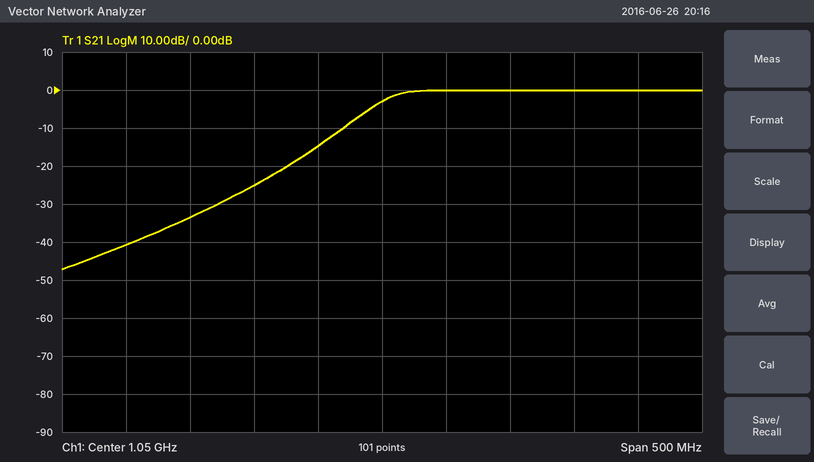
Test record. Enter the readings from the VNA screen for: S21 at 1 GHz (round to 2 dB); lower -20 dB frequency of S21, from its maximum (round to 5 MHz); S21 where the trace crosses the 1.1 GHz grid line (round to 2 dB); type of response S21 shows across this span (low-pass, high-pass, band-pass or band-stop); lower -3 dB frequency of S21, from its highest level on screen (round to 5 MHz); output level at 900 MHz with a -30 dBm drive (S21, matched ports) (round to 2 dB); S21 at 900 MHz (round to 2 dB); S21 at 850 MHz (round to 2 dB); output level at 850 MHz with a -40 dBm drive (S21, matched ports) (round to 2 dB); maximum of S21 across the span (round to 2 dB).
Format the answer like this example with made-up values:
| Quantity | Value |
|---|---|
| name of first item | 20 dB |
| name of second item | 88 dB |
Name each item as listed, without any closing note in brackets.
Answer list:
| Quantity | Value |
|---|---|
| S21 at 1 GHz | -14 dB |
| lower -20 dB frequency of S21, from its maximum | 975 MHz |
| S21 where the trace crosses the 1.1 GHz grid line | 0 dB |
| type of response S21 shows across this span | high-pass |
| lower -3 dB frequency of S21, from its highest level on screen | 1.050 GHz |
| output level at 900 MHz with a -30 dBm drive (S21, matched ports) | -64 dBm |
| S21 at 900 MHz | -34 dB |
| S21 at 850 MHz | -40 dB |
| output level at 850 MHz with a -40 dBm drive (S21, matched ports) | -80 dBm |
| maximum of S21 across the span | 0 dB |
